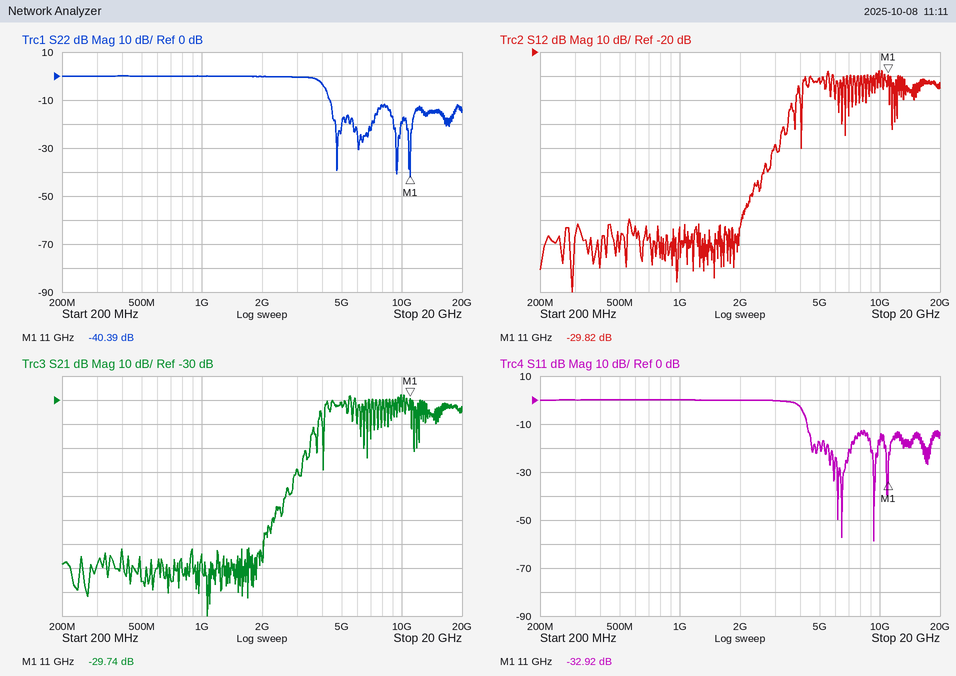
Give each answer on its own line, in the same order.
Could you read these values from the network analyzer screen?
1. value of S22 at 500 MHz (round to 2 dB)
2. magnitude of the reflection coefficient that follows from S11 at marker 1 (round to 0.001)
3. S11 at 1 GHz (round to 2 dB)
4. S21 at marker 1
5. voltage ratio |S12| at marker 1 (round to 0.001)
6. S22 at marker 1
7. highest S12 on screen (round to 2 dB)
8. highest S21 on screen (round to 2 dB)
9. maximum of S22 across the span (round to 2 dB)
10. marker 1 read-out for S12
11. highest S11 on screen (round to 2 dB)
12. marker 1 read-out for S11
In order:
0 dB
0.023
0 dB
-29.74 dB
0.032
-40.39 dB
-28 dB
-28 dB
0 dB
-29.82 dB
0 dB
-32.92 dB
